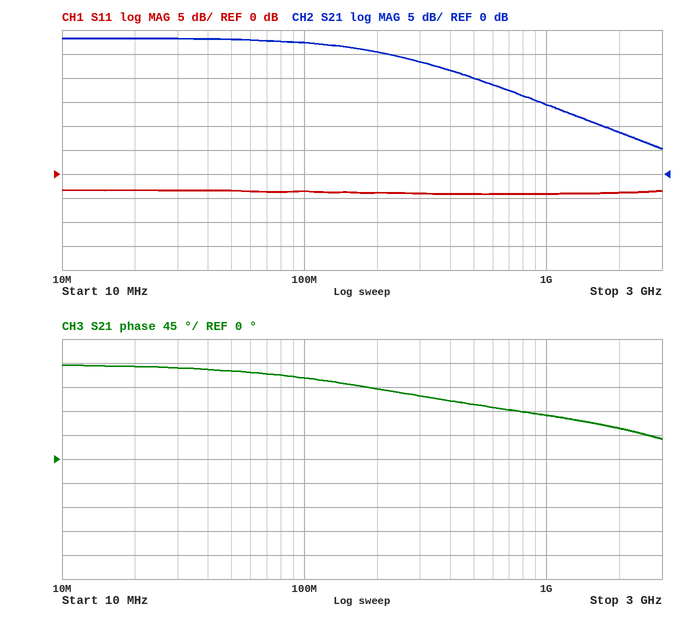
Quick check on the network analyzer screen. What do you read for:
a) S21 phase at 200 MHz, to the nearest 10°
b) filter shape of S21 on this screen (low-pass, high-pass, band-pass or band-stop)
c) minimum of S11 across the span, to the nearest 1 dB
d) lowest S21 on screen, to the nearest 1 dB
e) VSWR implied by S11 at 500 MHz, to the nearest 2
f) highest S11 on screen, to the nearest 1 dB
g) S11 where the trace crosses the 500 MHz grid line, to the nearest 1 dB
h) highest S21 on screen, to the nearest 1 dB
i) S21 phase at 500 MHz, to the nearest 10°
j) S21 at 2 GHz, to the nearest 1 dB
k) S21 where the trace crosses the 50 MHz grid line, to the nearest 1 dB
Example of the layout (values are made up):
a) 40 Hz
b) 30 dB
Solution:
a) 130°
b) low-pass
c) -4 dB
d) 5 dB
e) 4
f) -3 dB
g) -4 dB
h) 28 dB
i) 100°
j) 9 dB
k) 28 dB
